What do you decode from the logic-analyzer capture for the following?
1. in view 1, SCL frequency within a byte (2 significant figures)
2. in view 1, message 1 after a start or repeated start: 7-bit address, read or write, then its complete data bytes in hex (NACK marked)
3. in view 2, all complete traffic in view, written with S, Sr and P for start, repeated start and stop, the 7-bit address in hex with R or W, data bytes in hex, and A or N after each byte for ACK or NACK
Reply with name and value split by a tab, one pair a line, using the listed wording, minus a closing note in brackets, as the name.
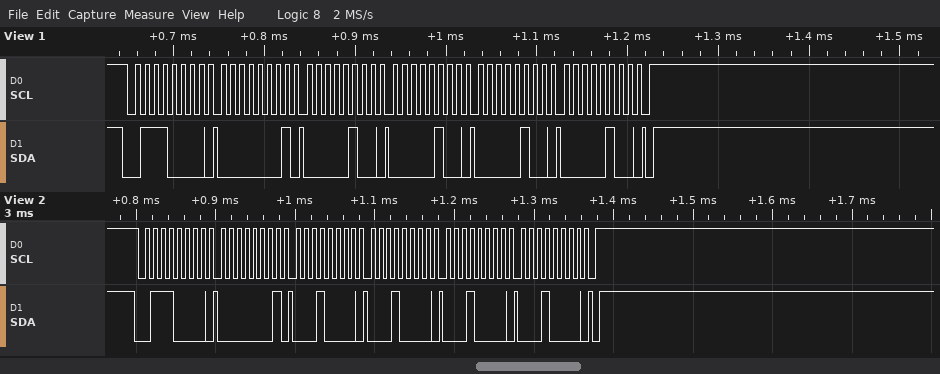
in view 1, SCL frequency within a byte	100 kHz
in view 1, message 1 after a start or repeated start: 7-bit address, read or write, then its complete data bytes in hex	0x38 write: 01 04 04 04 04
in view 2, all complete traffic in view, written with S, Sr and P for start, repeated start and stop, the 7-bit address in hex with R or W, data bytes in hex, and A or N after each byte for ACK or NACK	S 38W A 01 A 10 A 10 A 10 A 10 A P
